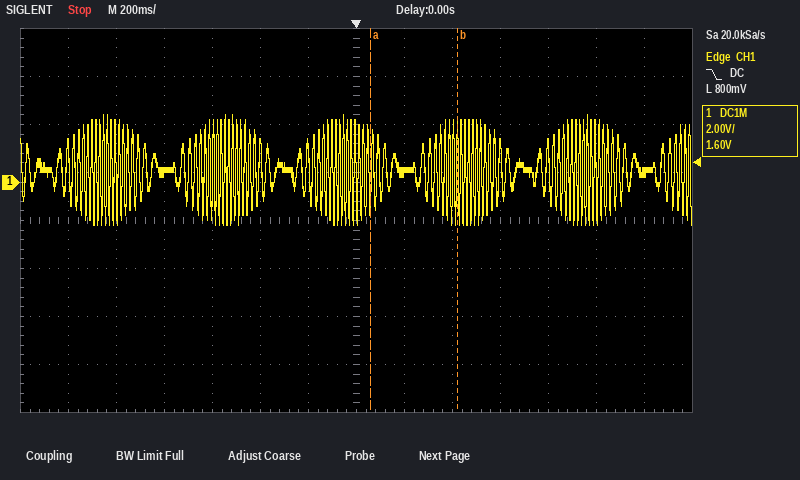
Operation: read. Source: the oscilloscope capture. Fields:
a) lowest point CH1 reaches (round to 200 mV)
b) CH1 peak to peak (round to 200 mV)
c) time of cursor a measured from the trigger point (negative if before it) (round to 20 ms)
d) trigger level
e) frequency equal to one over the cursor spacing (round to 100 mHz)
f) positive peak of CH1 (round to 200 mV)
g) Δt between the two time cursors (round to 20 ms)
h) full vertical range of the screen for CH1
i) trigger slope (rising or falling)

-1.8 V
4.6 V
+60 ms
800 mV
2.8 Hz
2.8 V
360 ms
16 V
falling
